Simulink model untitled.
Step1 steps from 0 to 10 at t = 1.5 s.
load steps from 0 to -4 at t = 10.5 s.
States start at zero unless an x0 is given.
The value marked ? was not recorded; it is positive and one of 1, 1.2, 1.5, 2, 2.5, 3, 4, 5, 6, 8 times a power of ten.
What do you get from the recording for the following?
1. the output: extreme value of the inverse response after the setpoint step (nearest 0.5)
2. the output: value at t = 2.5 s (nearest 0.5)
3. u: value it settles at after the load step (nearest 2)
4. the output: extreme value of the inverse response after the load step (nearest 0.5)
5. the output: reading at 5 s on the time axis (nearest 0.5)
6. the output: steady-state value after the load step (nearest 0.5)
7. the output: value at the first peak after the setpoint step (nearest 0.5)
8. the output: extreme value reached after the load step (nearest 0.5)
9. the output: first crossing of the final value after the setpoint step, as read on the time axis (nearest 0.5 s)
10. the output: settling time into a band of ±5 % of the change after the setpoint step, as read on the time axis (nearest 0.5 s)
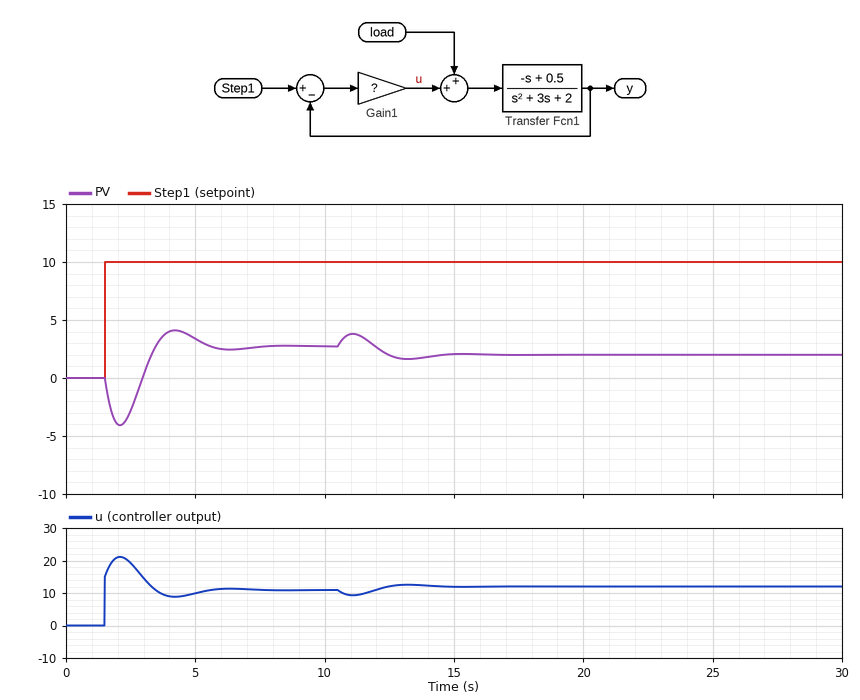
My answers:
-4.0
-3.0
12
4.0
3.5
2.0
4.0
1.5
3.5 s
7.0 s
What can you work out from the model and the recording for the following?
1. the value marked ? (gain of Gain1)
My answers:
1.5
